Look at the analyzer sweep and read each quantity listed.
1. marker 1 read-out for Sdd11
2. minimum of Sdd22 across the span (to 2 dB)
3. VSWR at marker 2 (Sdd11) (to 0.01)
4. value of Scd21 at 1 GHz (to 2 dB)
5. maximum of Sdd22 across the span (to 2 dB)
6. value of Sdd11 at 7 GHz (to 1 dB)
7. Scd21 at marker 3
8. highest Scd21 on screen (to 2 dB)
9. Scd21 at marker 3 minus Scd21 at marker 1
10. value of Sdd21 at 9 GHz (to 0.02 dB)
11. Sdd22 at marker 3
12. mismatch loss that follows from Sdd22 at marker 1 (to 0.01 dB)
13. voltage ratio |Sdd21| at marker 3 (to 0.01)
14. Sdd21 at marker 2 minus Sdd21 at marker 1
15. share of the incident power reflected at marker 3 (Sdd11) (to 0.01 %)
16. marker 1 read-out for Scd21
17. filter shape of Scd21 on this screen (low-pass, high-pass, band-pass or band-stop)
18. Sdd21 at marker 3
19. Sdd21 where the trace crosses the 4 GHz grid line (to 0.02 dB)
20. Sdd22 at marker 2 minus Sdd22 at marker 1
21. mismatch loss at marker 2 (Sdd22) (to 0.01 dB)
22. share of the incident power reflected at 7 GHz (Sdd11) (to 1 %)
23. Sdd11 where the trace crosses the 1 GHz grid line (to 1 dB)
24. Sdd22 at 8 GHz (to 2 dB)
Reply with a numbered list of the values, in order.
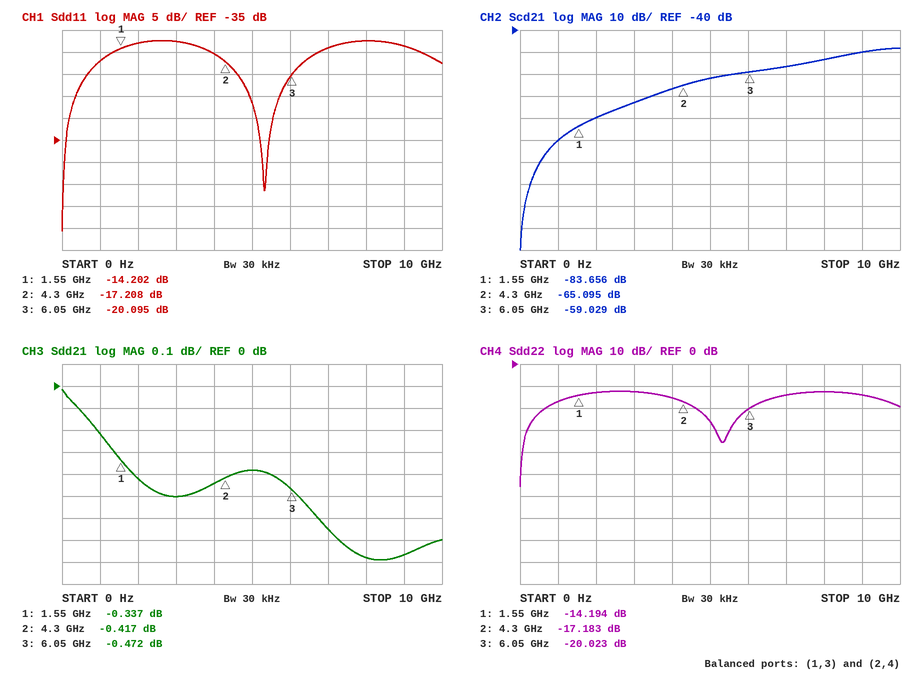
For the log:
1. -14.202 dB
2. -56 dB
3. 1.32
4. -90 dB
5. -12 dB
6. -14 dB
7. -59.029 dB
8. -48 dB
9. 24.627 dB
10. -0.76 dB
11. -20.023 dB
12. 0.17 dB
13. 0.95
14. -0.080 dB
15. 0.98 %
16. -83.656 dB
17. high-pass
18. -0.472 dB
19. -0.44 dB
20. -2.989 dB
21. 0.08 dB
22. 4 %
23. -17 dB
24. -12 dB
